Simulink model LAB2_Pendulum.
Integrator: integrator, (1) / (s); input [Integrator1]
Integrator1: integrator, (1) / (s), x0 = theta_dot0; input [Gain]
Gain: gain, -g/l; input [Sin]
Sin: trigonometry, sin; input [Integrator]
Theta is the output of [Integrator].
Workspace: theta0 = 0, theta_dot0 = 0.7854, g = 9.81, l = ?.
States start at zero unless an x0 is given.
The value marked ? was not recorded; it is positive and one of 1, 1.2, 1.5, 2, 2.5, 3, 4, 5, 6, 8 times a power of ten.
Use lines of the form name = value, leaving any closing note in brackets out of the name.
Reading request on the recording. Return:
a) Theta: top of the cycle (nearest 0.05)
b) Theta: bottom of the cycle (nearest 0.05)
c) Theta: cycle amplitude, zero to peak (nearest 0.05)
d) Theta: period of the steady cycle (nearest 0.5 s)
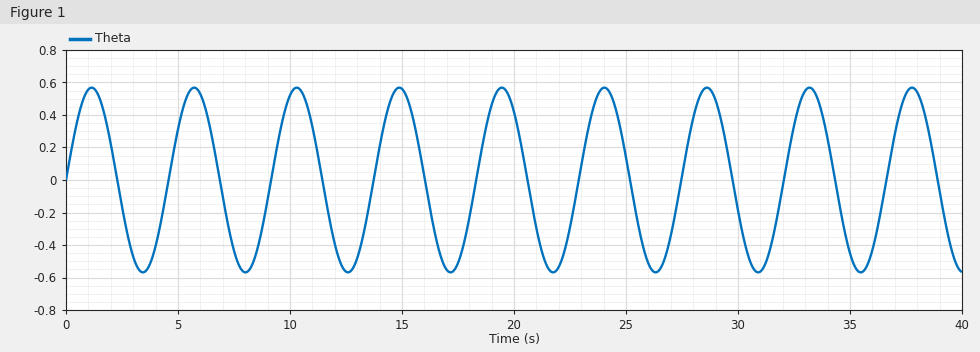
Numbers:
Theta: top of the cycle = 0.55
Theta: bottom of the cycle = -0.55
Theta: cycle amplitude, zero to peak = 0.55
Theta: period of the steady cycle = 4.5 s
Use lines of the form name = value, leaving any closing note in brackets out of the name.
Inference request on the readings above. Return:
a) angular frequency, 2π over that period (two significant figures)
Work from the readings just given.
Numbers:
angular frequency, 2π over that period = 1.4 rad/s
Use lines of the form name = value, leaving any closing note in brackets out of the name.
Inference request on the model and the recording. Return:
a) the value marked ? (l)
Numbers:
the value marked ? = 5
